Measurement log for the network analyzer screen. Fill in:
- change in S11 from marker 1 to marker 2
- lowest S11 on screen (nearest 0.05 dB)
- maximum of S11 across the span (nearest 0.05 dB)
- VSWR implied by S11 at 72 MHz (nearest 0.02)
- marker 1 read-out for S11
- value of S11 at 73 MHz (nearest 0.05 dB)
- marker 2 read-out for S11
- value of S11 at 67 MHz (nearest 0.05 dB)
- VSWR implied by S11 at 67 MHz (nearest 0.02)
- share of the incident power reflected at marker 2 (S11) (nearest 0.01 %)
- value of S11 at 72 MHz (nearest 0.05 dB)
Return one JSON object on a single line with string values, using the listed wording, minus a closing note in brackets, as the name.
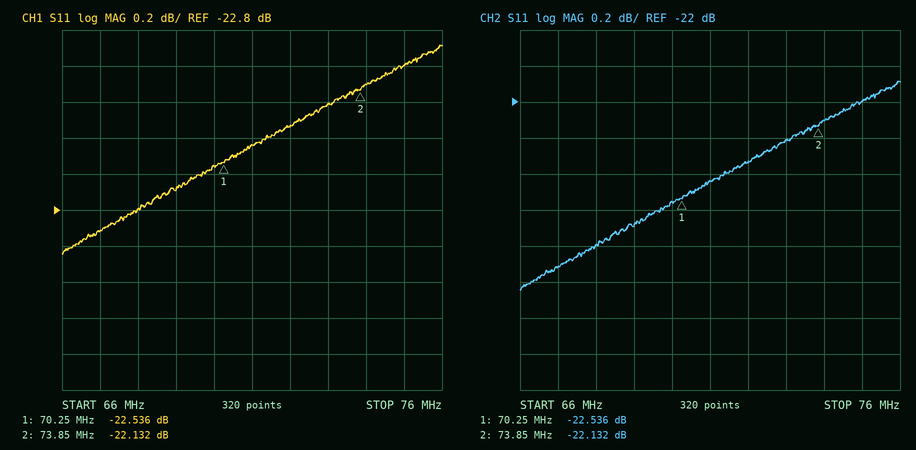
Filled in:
{"change in S11 from marker 1 to marker 2": "0.404 dB", "lowest S11 on screen": "-23.05 dB", "maximum of S11 across the span": "-21.90 dB", "VSWR implied by S11 at 72 MHz": "1.16", "marker 1 read-out for S11": "-22.536 dB", "value of S11 at 73 MHz": "-22.20 dB", "marker 2 read-out for S11": "-22.132 dB", "value of S11 at 67 MHz": "-22.90 dB", "VSWR implied by S11 at 67 MHz": "1.16", "share of the incident power reflected at marker 2 (S11)": "0.61 %", "value of S11 at 72 MHz": "-22.35 dB"}
